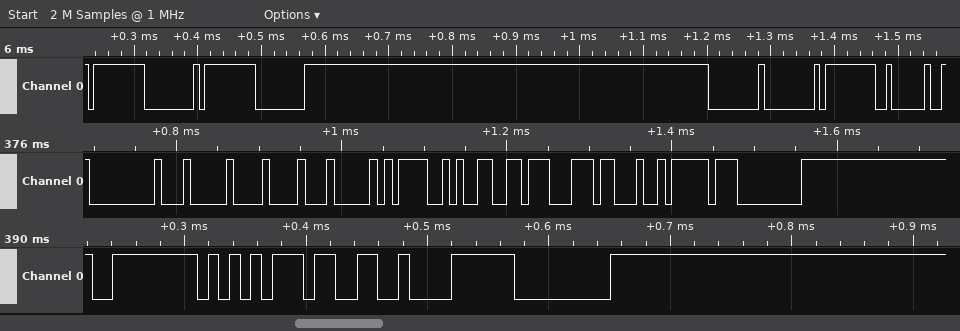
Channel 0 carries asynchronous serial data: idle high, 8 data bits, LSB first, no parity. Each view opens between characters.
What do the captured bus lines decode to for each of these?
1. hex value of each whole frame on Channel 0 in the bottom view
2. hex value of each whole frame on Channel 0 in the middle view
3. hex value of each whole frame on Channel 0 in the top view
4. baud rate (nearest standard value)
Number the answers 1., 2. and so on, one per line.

1. FE, D5, 33, F8, 00
2. 00, 04, 08, 04, 3D, 99, C7, 23, DF, 00
3. FF, 00, FF, 00, 00, 00, FF, 02
4. 115200 baud
